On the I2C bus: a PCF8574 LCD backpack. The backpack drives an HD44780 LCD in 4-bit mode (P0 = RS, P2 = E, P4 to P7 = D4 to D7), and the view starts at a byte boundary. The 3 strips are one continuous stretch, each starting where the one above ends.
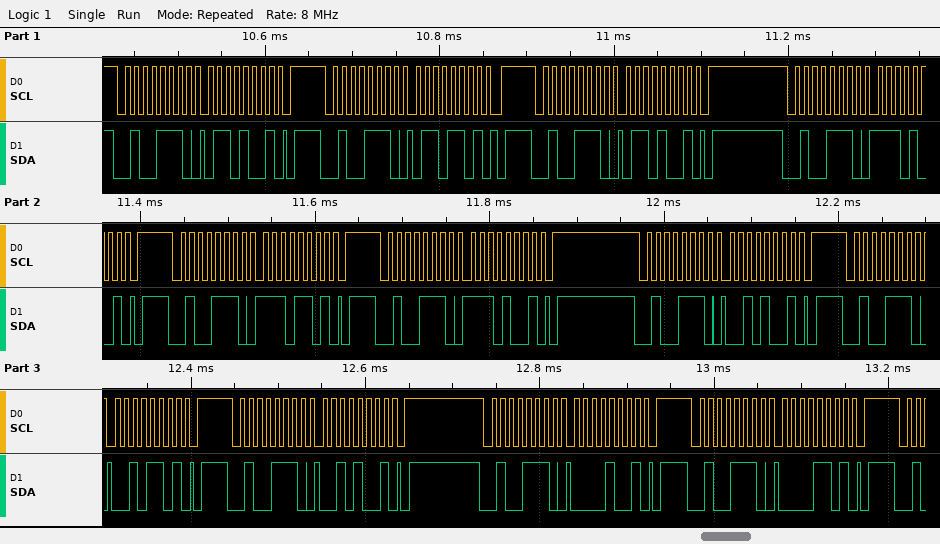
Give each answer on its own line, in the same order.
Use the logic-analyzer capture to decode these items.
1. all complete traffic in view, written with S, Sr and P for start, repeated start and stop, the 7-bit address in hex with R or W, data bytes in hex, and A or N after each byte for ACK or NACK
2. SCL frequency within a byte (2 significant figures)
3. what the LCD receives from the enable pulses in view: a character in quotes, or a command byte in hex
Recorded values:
S 27W A 69 A P S 27W A 6D A P S 27W A 69 A P S 27W A E9 A P S 27W A ED A P S 27W A E9 A P S 27W A 29 A P S 27W A 2D A P S 27W A 29 A P S 27W A 09 A P S 27W A 0D A P
100 kHz
'n'
